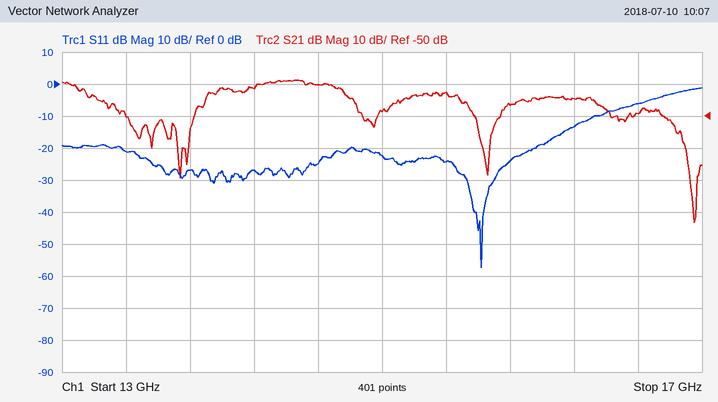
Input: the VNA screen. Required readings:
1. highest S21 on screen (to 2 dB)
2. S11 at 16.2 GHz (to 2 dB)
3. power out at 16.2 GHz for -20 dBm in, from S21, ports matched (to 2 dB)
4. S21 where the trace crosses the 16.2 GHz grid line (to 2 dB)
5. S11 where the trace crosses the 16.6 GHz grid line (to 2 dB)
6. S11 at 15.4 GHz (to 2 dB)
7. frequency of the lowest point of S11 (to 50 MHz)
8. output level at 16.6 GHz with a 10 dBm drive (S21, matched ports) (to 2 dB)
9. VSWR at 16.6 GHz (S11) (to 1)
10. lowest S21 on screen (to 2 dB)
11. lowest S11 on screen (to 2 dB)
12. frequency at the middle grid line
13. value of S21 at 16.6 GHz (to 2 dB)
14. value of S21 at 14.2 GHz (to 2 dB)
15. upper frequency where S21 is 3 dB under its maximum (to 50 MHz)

-38 dB
-14 dB
-64 dBm
-44 dB
-6 dB
-24 dB
15.60 GHz
-40 dBm
3
-84 dB
-58 dB
15 GHz
-50 dB
-42 dB
14.75 GHz
